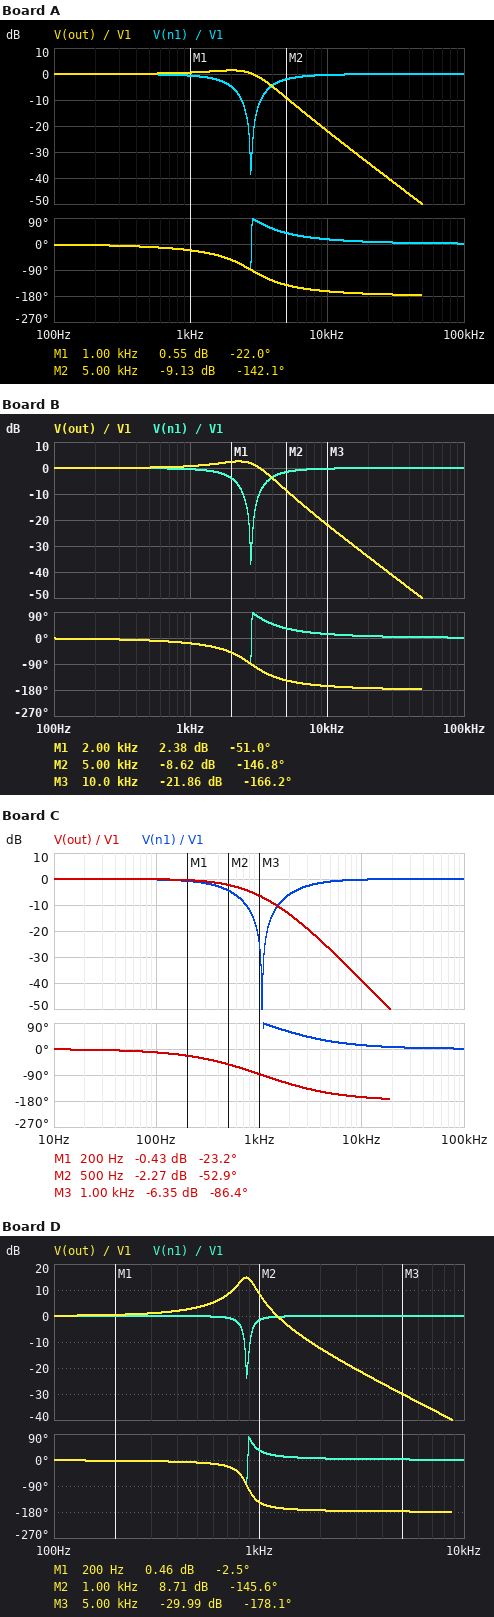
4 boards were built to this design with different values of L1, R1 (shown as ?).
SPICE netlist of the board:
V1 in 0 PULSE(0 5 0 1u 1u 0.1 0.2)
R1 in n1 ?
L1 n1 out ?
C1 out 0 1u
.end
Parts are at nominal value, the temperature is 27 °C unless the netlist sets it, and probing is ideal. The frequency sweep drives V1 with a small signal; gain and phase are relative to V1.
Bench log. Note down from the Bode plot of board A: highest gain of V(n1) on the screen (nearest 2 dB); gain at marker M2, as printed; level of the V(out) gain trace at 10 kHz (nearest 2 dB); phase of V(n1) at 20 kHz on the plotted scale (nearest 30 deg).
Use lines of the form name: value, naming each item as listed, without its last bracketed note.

highest gain of V(n1) on the screen: 0 dB
gain at marker M2, as printed: -9.13 dB
level of the V(out) gain trace at 10 kHz: -22 dB
phase of V(n1) at 20 kHz on the plotted scale: 0 deg
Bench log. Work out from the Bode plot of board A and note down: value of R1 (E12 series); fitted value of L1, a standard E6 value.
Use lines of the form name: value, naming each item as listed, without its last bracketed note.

value of R1: 56 Ω
fitted value of L1, a standard E6 value: 3.3 mH
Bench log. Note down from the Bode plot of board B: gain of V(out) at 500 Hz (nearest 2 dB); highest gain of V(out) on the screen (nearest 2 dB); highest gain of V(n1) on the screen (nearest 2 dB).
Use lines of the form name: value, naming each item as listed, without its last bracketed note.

gain of V(out) at 500 Hz: 0 dB
highest gain of V(out) on the screen: 2 dB
highest gain of V(n1) on the screen: 0 dB
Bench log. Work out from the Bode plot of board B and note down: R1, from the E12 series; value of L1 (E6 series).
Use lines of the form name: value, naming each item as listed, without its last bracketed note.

R1, from the E12 series: 47 Ω
value of L1: 3.3 mH
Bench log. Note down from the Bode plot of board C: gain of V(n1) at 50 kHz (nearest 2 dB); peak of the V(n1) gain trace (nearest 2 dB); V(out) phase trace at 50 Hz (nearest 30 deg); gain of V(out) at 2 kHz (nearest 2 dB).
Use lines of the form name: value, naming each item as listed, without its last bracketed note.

gain of V(n1) at 50 kHz: 0 dB
peak of the V(n1) gain trace: 0 dB
V(out) phase trace at 50 Hz: 0 deg
gain of V(out) at 2 kHz: -14 dB
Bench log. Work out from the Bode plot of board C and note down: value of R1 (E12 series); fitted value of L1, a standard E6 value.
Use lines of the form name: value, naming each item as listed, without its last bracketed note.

value of R1: 330 Ω
fitted value of L1, a standard E6 value: 22 mH
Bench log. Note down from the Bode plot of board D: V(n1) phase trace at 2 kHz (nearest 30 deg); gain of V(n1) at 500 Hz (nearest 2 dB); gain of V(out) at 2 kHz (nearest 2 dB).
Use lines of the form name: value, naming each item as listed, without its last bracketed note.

V(n1) phase trace at 2 kHz: 0 deg
gain of V(n1) at 500 Hz: 0 dB
gain of V(out) at 2 kHz: -12 dB
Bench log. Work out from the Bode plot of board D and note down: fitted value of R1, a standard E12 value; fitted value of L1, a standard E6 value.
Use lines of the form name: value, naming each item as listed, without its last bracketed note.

fitted value of R1, a standard E12 value: 33 Ω
fitted value of L1, a standard E6 value: 33 mH
